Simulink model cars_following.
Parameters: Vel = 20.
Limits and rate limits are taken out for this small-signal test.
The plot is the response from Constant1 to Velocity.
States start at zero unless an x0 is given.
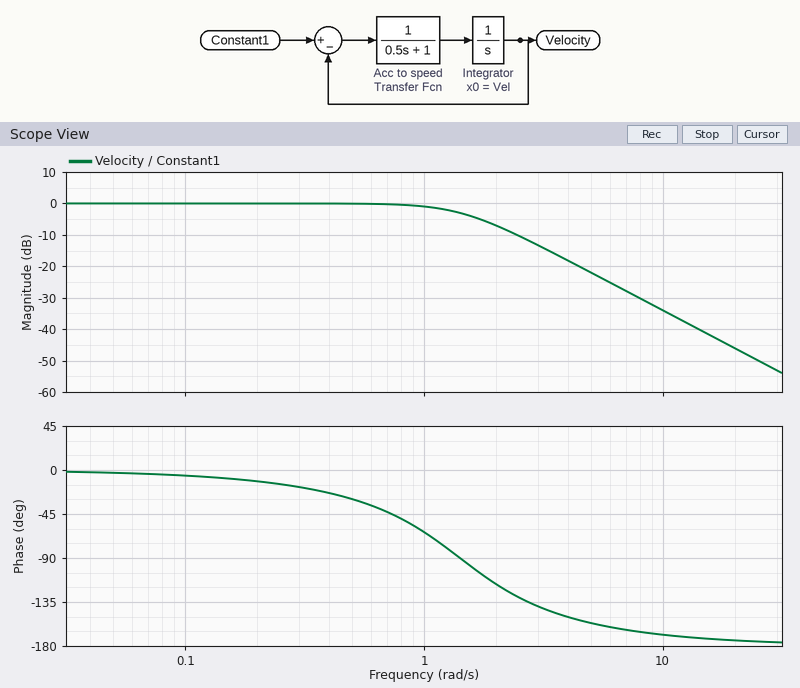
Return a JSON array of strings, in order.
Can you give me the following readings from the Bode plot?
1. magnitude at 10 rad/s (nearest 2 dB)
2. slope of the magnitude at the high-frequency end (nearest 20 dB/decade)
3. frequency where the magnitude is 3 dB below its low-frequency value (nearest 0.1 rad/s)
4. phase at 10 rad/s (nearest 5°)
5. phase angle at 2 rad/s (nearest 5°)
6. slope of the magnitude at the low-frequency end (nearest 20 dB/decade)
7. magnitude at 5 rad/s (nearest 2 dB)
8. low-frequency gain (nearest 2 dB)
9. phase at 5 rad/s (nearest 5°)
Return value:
["-34 dB", "-40 dB/decade", "1.4 rad/s", "-170°", "-115°", "0 dB/decade", "-22 dB", "0 dB", "-155°"]
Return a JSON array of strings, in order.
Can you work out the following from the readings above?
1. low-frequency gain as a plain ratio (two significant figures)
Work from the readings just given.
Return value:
["1.0"]
